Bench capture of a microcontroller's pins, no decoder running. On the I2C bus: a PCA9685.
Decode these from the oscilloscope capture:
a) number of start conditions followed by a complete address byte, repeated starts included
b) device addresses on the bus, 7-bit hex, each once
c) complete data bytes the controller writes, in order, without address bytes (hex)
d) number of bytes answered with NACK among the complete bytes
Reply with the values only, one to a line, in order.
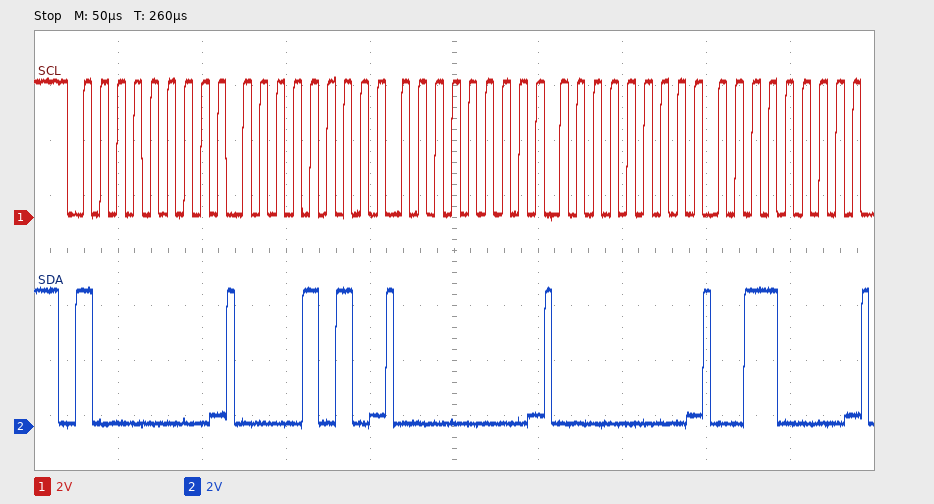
1
0x40
0A 00 00 30
0
